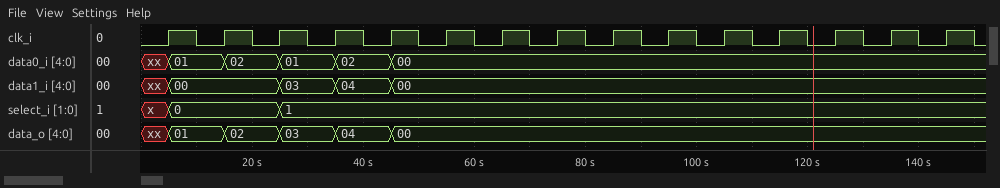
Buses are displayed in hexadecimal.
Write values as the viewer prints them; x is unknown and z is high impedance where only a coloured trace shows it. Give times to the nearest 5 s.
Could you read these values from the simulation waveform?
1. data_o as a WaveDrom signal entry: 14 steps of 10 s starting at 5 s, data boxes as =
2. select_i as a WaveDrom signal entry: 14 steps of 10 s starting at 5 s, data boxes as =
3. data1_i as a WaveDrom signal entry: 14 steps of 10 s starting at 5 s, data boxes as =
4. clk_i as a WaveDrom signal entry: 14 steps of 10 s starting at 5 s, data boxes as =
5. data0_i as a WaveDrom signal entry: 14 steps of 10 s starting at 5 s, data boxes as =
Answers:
{name: 'data_o', wave: '=====.........', data: '01 02 03 04 00'}
{name: 'select_i', wave: '=.=...........', data: '0 1'}
{name: 'data1_i', wave: '=.===.........', data: '00 03 04 00'}
{name: 'clk_i', wave: 'p.............'}
{name: 'data0_i', wave: '=====.........', data: '01 02 01 02 00'}
